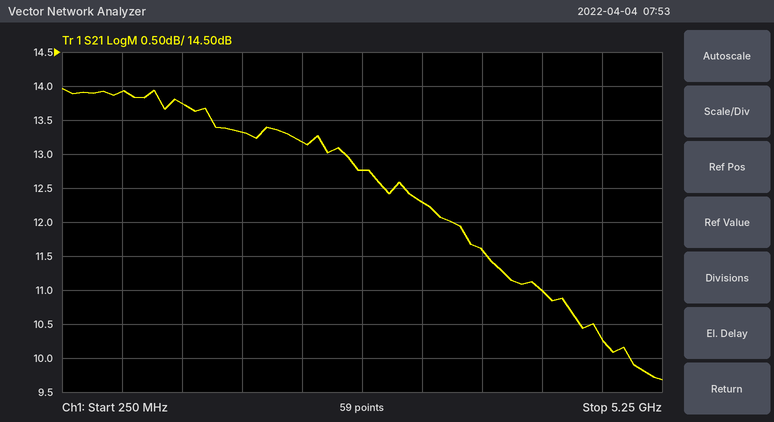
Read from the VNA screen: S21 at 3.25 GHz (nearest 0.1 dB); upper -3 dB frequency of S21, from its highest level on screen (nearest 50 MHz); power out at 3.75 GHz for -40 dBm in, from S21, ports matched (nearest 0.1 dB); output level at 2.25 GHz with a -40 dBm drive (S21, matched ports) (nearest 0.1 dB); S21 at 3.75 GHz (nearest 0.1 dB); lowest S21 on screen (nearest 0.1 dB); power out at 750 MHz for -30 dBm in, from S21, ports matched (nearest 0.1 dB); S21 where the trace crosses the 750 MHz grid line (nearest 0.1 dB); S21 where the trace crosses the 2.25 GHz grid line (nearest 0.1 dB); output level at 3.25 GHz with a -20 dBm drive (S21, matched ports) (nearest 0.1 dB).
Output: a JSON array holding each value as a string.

["12.3 dB", "4.25 GHz", "-28.4 dBm", "-26.8 dBm", "11.6 dB", "9.7 dB", "-16.1 dBm", "13.9 dB", "13.2 dB", "-7.7 dBm"]
